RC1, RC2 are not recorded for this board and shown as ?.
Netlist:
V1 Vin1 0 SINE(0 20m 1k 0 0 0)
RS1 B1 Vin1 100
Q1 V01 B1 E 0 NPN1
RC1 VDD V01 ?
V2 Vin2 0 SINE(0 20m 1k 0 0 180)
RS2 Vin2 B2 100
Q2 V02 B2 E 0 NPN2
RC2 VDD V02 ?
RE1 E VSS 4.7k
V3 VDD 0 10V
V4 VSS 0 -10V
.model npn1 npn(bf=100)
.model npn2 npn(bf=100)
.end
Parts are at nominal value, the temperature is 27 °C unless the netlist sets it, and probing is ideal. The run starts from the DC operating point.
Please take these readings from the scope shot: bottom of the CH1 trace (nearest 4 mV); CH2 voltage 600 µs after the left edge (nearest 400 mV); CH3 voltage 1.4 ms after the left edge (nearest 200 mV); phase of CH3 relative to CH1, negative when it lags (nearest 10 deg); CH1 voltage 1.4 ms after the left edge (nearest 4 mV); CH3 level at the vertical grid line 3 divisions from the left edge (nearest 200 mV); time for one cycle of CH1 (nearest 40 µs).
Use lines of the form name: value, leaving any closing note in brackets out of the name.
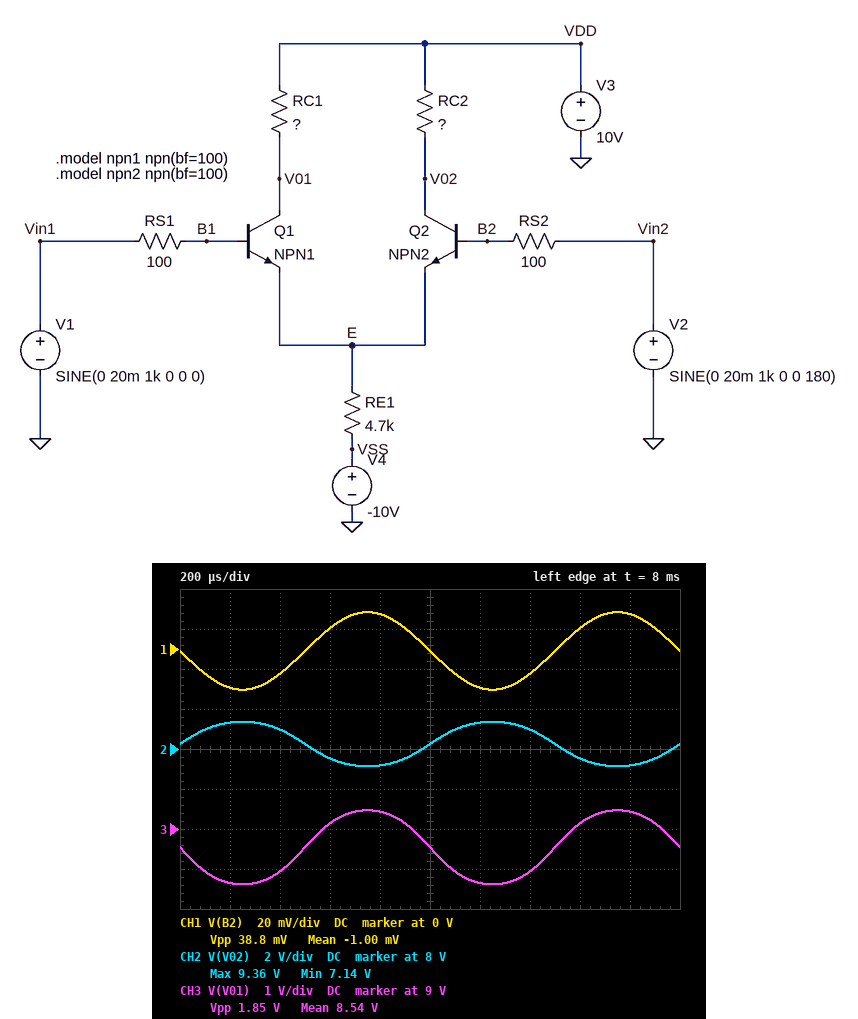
bottom of the CH1 trace: -20 mV
CH2 voltage 600 µs after the left edge: 7.6 V
CH3 voltage 1.4 ms after the left edge: 8.0 V
phase of CH3 relative to CH1, negative when it lags: 0 deg
CH1 voltage 1.4 ms after the left edge: -12 mV
CH3 level at the vertical grid line 3 divisions from the left edge: 9.2 V
time for one cycle of CH1: 1.00 ms
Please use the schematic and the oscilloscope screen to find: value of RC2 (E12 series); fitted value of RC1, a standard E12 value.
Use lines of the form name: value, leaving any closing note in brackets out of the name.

value of RC2: 1.8 kΩ
fitted value of RC1, a standard E12 value: 1.5 kΩ
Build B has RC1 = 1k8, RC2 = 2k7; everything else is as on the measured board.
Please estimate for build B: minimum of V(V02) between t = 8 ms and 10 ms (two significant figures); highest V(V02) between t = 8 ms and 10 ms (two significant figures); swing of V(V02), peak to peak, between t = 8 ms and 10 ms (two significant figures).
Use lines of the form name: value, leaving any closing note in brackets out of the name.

minimum of V(V02) between t = 8 ms and 10 ms: 5.7 V
highest V(V02) between t = 8 ms and 10 ms: 9.0 V
swing of V(V02), peak to peak, between t = 8 ms and 10 ms: 3.3 V
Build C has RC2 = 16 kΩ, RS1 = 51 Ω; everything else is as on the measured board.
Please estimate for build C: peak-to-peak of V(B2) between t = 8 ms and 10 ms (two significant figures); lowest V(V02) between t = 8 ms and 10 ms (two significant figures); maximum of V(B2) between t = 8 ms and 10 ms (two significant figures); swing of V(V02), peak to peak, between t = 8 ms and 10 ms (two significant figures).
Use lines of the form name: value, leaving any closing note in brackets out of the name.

peak-to-peak of V(B2) between t = 8 ms and 10 ms: 11 mV
lowest V(V02) between t = 8 ms and 10 ms: -760 mV
maximum of V(B2) between t = 8 ms and 10 ms: -9.1 mV
swing of V(V02), peak to peak, between t = 8 ms and 10 ms: 5.2 V
